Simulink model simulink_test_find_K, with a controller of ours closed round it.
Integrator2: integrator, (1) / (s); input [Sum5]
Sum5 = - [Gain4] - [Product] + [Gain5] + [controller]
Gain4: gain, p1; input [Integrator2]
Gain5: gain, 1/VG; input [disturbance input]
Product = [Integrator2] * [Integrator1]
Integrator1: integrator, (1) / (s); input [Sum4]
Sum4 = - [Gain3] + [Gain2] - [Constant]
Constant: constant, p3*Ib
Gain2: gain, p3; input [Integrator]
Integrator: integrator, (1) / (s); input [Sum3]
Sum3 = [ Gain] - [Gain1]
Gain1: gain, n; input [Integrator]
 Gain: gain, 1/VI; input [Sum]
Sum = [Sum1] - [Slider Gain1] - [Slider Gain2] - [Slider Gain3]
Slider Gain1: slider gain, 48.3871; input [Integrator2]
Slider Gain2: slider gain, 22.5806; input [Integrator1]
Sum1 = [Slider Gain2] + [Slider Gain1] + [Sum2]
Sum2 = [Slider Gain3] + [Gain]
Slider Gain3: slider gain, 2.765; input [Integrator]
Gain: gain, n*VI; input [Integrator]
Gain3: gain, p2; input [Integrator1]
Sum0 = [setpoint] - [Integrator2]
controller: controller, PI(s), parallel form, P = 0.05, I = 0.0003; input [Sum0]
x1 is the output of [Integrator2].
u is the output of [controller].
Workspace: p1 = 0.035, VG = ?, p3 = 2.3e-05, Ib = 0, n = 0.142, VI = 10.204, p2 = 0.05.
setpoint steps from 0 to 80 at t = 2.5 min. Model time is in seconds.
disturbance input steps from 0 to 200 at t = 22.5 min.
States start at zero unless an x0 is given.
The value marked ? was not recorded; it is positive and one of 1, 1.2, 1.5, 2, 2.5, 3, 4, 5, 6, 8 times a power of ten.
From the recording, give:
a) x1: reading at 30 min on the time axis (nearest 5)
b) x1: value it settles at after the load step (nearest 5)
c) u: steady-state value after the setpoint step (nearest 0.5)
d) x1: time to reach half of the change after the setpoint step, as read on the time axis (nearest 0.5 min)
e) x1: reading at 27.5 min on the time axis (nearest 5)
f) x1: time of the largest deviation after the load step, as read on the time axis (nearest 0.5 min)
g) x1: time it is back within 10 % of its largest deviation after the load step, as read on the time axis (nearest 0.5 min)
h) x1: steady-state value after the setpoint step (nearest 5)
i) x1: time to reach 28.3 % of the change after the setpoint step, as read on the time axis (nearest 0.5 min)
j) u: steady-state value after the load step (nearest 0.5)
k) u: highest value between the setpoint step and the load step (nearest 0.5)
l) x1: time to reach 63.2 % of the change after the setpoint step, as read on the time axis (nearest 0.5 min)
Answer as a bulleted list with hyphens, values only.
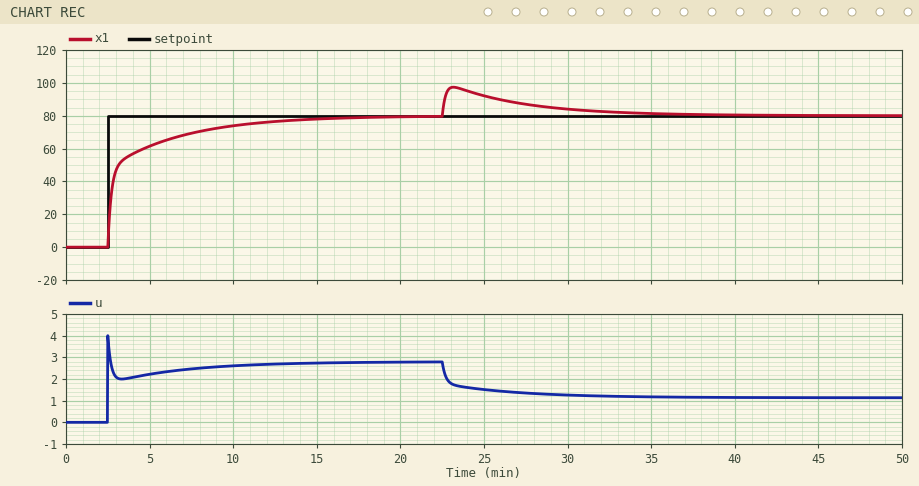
- 85
- 80
- 3.0
- 3.0 min
- 85
- 23.0 min
- 33.5 min
- 80
- 2.5 min
- 1.0
- 4.0
- 3.0 min
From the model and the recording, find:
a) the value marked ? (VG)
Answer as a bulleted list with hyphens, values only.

- 120
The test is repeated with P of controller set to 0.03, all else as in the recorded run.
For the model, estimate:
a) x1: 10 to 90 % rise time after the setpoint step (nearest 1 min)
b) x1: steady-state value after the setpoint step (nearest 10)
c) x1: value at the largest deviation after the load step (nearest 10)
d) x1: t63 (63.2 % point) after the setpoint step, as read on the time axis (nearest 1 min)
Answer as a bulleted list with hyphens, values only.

- 6 min
- 80
- 100
- 4 min
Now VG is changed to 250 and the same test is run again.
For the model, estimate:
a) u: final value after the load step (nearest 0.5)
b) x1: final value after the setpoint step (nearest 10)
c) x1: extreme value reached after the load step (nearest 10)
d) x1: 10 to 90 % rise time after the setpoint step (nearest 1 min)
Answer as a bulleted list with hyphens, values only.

- 2.0
- 80
- 90
- 6 min
